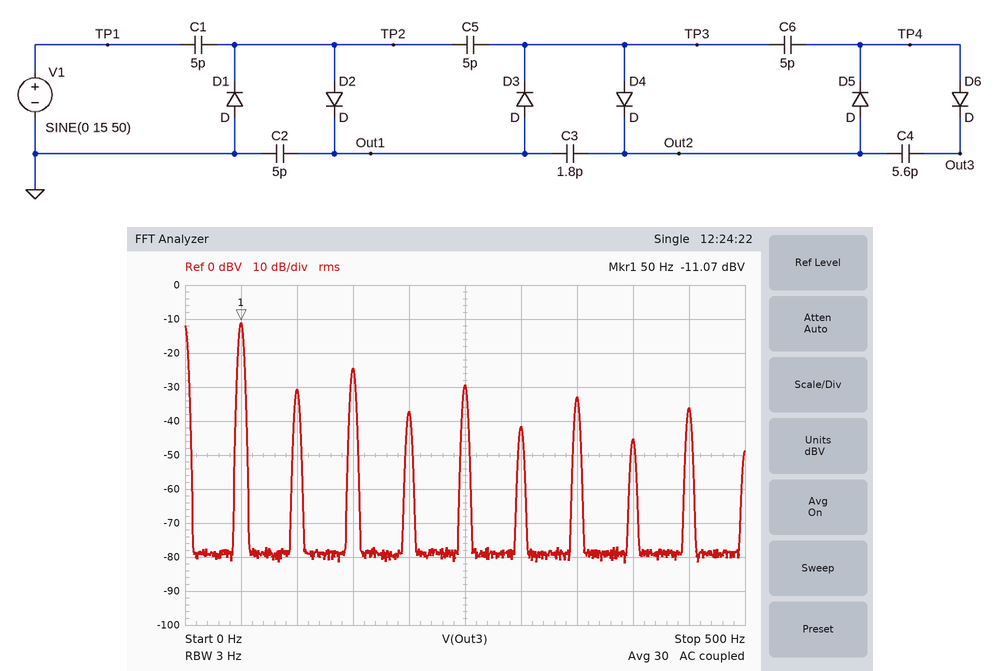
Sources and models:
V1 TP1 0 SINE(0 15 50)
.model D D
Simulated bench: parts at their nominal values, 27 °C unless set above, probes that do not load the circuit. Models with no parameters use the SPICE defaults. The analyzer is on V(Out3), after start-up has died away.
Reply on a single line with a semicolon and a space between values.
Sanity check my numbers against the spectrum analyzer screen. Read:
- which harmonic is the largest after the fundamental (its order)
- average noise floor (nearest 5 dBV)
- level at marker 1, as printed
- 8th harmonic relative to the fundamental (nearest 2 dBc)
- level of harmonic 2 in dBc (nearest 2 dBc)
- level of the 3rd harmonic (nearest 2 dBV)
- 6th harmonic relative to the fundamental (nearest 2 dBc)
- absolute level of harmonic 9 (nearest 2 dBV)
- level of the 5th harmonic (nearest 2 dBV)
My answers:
3; -80 dBV; -11.07 dBV; -34 dBc; -20 dBc; -24 dBV; -30 dBc; -36 dBV; -30 dBV
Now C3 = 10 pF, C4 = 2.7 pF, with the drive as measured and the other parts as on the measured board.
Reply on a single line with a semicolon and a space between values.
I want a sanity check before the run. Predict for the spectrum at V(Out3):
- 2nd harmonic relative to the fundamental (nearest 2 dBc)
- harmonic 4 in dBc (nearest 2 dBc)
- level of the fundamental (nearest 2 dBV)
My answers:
-18 dBc; -24 dBc; -16 dBV
